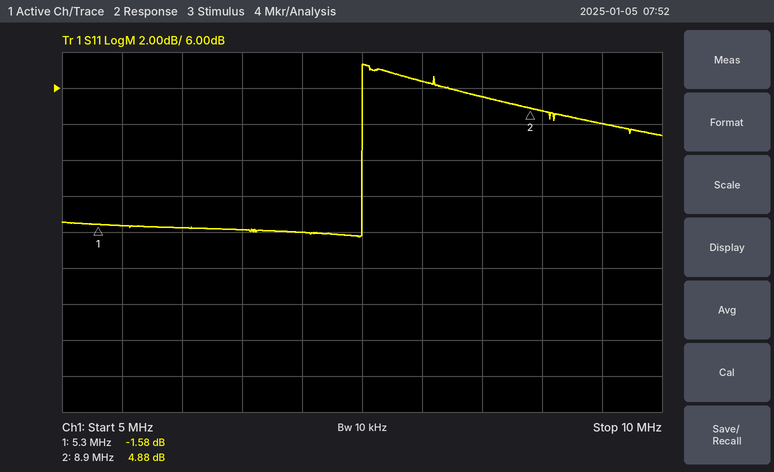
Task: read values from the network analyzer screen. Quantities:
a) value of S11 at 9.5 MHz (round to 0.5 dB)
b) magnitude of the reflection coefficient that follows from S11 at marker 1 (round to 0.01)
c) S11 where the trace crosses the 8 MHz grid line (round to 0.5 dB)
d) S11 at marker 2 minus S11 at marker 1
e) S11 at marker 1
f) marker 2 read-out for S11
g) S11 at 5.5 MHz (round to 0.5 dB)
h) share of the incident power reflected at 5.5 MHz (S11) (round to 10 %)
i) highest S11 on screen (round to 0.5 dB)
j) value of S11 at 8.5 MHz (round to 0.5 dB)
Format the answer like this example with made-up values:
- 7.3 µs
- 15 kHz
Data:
- 4.0 dB
- 0.83
- 6.5 dB
- 6.46 dB
- -1.58 dB
- 4.88 dB
- -1.5 dB
- 70 %
- 7.5 dB
- 5.5 dB
